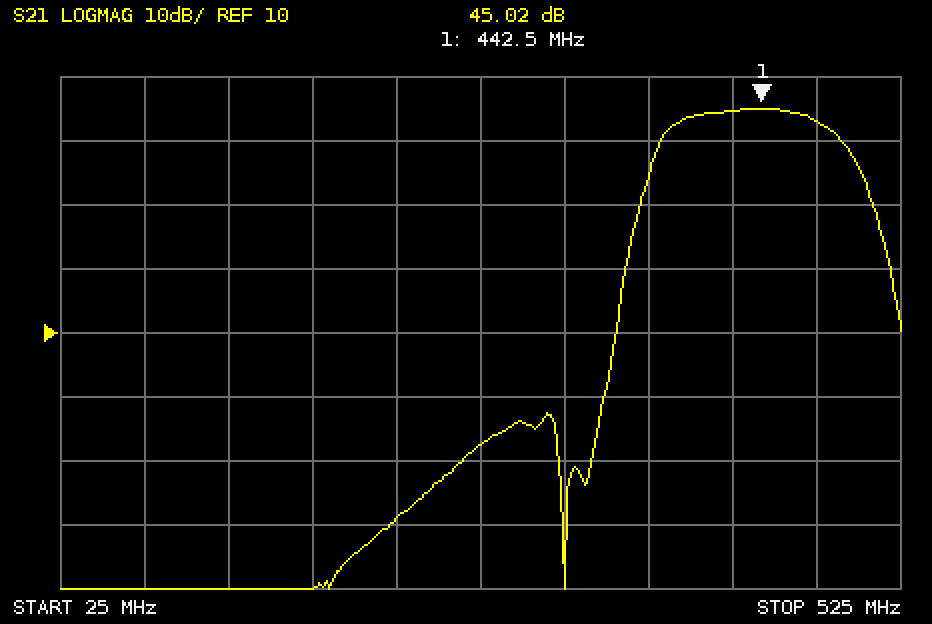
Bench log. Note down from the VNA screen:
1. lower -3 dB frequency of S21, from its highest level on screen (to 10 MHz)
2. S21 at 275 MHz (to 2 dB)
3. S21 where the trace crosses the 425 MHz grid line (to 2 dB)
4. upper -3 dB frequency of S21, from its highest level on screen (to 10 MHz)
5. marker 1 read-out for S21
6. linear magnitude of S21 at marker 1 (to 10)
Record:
390 MHz
-8 dB
44 dB
480 MHz
45.02 dB
180
